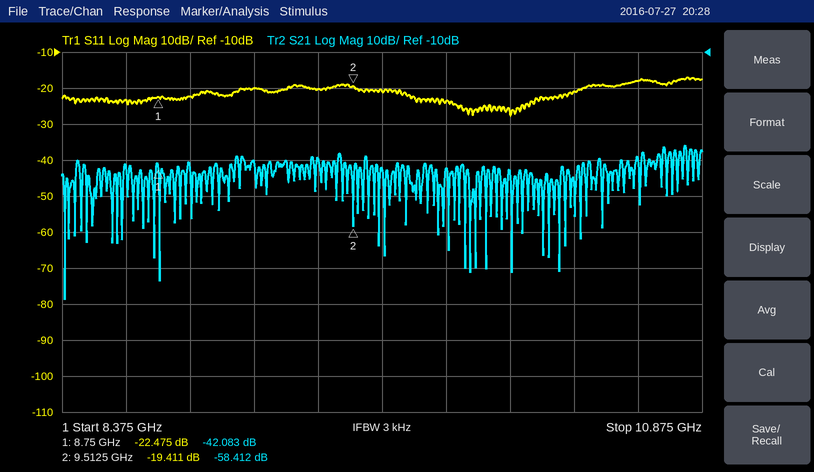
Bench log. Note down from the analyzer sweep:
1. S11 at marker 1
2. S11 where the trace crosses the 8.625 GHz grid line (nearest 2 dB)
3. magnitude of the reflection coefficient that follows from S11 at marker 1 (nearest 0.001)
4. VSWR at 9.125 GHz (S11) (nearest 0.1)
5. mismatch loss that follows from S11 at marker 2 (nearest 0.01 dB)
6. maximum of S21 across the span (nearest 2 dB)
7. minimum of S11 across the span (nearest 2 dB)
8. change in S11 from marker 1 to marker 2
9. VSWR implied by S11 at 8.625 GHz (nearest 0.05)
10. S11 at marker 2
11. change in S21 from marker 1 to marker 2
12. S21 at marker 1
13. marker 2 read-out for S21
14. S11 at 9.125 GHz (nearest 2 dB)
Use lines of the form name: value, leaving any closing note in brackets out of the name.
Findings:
S11 at marker 1: -22.475 dB
S11 where the trace crosses the 8.625 GHz grid line: -24 dB
magnitude of the reflection coefficient that follows from S11 at marker 1: 0.075
VSWR at 9.125 GHz (S11): 1.2
mismatch loss that follows from S11 at marker 2: 0.05 dB
maximum of S21 across the span: -36 dB
minimum of S11 across the span: -28 dB
change in S11 from marker 1 to marker 2: 3.064 dB
VSWR implied by S11 at 8.625 GHz: 1.15
S11 at marker 2: -19.411 dB
change in S21 from marker 1 to marker 2: -16.329 dB
S21 at marker 1: -42.083 dB
marker 2 read-out for S21: -58.412 dB
S11 at 9.125 GHz: -20 dB
